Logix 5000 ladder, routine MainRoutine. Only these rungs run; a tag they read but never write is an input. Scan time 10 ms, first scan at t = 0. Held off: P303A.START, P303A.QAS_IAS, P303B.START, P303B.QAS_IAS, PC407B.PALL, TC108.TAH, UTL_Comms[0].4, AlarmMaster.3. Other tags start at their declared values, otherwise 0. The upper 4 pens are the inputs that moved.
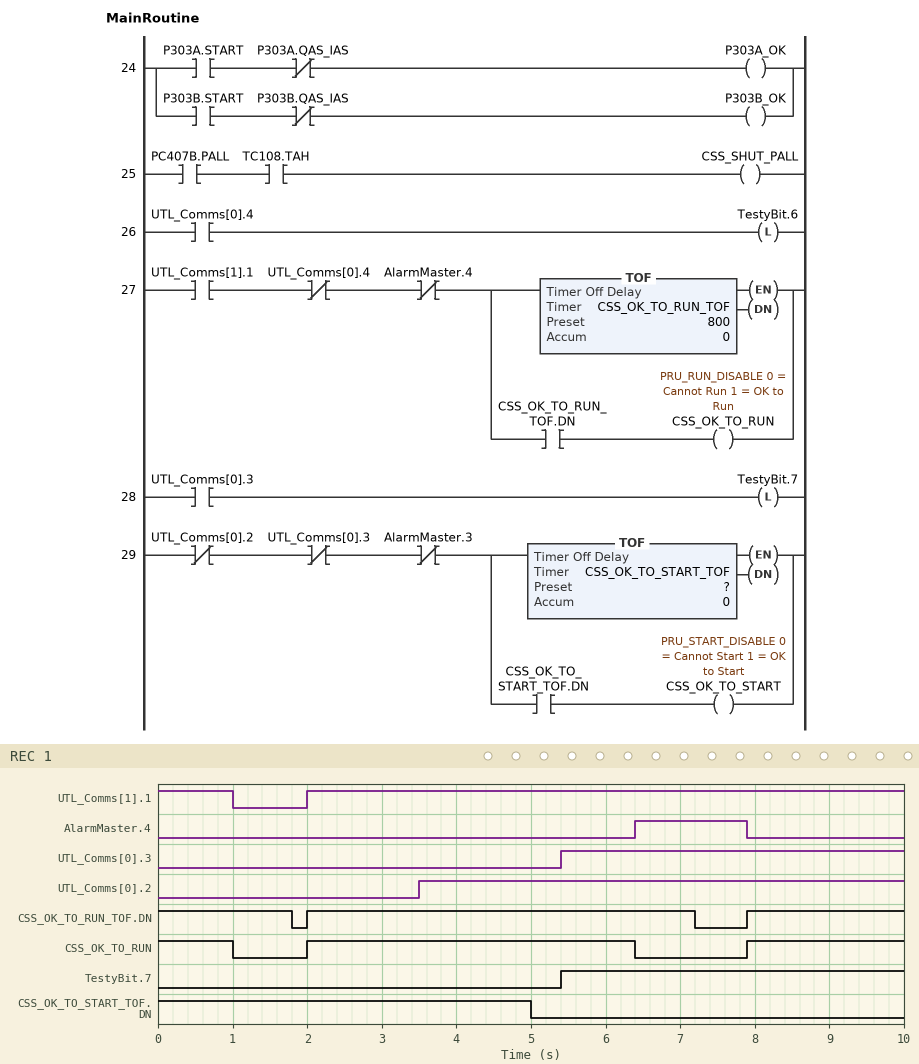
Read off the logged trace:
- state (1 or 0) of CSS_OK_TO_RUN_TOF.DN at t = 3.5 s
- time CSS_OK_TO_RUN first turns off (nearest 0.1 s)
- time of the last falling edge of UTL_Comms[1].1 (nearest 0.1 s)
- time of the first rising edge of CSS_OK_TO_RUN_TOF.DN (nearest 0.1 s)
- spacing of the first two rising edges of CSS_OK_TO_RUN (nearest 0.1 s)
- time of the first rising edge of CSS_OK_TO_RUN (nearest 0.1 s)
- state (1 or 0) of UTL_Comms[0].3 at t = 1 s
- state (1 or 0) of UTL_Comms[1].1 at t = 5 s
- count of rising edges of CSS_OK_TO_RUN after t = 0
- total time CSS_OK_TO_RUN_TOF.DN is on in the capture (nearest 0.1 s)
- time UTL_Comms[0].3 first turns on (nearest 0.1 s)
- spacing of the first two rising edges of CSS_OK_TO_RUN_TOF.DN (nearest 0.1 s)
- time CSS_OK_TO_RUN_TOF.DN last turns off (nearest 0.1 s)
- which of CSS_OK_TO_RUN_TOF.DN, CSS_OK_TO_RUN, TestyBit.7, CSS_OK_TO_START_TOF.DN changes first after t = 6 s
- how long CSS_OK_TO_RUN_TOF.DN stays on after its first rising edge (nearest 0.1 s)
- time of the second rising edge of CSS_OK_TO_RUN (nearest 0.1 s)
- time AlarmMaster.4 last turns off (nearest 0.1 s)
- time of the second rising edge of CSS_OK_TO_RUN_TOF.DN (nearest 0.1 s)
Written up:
1
1.0 s
1.0 s
2.0 s
5.9 s
2.0 s
0
1
2
9.1 s
5.4 s
5.9 s
7.2 s
CSS_OK_TO_RUN
5.2 s
7.9 s
7.9 s
7.9 s
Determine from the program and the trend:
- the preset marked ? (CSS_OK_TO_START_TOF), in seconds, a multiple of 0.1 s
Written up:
1.5 s
